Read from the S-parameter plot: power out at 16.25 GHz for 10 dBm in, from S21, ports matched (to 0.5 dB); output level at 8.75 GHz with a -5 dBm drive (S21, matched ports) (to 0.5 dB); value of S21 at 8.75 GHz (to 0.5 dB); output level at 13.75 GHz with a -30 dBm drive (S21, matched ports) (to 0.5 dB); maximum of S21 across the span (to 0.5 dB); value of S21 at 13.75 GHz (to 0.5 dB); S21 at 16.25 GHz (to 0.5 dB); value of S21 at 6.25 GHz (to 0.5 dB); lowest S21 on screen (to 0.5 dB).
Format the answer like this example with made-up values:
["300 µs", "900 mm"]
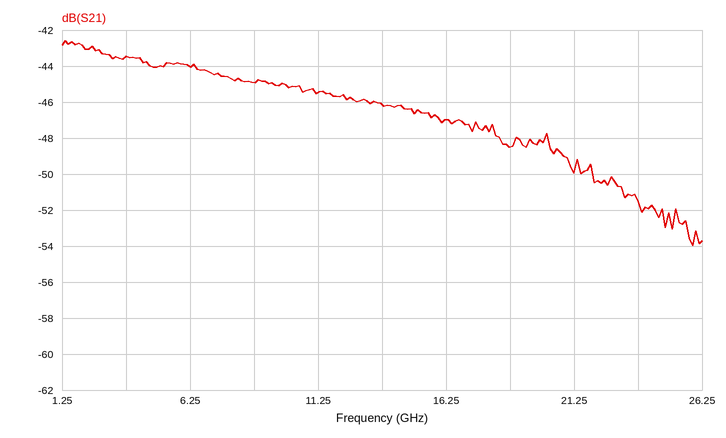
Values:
["-37.0 dBm", "-50.0 dBm", "-45.0 dB", "-76.0 dBm", "-42.5 dB", "-46.0 dB", "-47.0 dB", "-44.0 dB", "-54.0 dB"]
